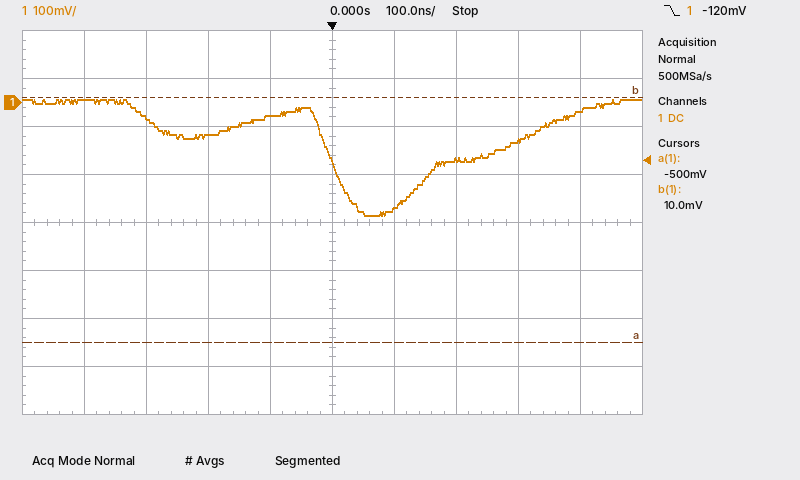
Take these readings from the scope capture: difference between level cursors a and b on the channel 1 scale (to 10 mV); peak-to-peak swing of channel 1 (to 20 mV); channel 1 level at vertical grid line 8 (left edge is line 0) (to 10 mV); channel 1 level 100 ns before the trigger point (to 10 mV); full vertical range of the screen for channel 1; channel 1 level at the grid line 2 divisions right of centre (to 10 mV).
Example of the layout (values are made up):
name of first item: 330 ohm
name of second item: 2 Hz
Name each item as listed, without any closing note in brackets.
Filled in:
difference between level cursors a and b on the channel 1 scale: 510 mV
peak-to-peak swing of channel 1: 240 mV
channel 1 level at vertical grid line 8 (left edge is line 0): -80 mV
channel 1 level 100 ns before the trigger point: -30 mV
full vertical range of the screen for channel 1: 800 mV
channel 1 level at the grid line 2 divisions right of centre: -120 mV
